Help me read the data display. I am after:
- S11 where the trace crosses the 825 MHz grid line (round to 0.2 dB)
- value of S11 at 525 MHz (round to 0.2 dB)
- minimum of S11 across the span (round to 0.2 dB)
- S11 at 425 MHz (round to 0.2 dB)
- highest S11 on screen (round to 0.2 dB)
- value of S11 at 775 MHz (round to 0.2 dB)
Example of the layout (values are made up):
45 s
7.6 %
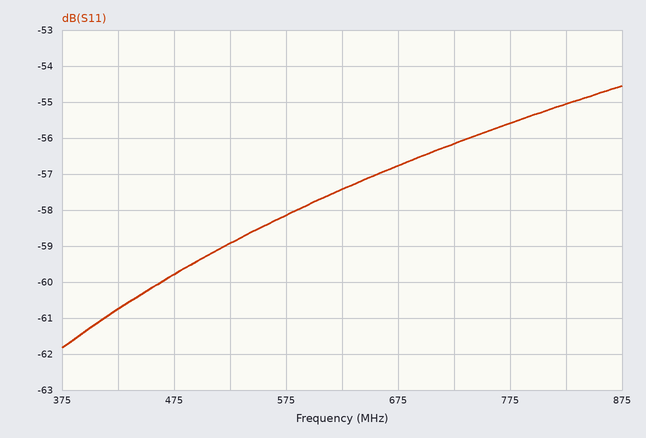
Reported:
-55.0 dB
-59.0 dB
-61.8 dB
-60.8 dB
-54.6 dB
-55.6 dB
